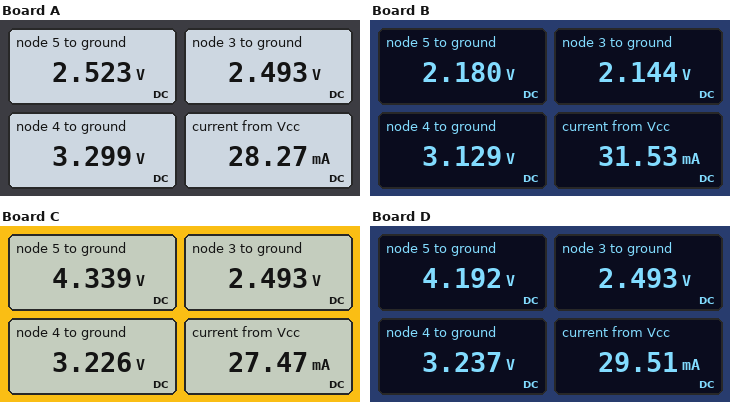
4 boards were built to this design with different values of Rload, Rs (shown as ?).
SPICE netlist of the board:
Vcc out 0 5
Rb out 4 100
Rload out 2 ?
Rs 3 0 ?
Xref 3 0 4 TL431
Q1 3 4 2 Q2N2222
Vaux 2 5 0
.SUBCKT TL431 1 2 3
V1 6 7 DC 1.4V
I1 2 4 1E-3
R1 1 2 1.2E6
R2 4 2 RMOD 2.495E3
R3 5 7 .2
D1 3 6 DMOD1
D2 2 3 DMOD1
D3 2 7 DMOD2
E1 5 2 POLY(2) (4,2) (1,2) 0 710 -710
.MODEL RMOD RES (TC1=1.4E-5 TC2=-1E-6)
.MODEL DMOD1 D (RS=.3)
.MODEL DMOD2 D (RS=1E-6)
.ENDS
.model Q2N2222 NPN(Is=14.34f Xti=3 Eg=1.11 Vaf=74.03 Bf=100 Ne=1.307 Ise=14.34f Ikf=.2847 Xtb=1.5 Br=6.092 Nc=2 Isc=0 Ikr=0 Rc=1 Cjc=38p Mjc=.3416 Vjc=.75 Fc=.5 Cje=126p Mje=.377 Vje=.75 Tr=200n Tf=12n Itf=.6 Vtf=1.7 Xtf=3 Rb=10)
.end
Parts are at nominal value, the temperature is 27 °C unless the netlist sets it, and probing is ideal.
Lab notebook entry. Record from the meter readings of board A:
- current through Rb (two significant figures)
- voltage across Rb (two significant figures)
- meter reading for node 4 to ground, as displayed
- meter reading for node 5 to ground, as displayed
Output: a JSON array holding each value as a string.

["17 mA", "1.7 V", "3.299 V", "2.523 V"]
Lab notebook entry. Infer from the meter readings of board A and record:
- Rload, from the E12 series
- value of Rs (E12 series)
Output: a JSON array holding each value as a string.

["220 Ω", "150 Ω"]
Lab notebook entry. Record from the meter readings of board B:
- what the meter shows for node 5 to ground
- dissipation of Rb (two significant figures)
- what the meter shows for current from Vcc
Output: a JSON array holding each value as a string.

["2.180 V", "35 mW", "31.53 mA"]
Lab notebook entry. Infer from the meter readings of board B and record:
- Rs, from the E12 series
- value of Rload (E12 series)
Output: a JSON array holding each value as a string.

["68 Ω", "220 Ω"]
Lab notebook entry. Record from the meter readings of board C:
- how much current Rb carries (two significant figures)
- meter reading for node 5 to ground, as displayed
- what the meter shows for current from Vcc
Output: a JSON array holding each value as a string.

["18 mA", "4.339 V", "27.47 mA"]
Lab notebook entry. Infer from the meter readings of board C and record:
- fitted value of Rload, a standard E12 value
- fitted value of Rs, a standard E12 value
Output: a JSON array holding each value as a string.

["68 Ω", "220 Ω"]
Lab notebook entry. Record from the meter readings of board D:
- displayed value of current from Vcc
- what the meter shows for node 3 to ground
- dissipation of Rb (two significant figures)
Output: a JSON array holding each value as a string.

["29.51 mA", "2.493 V", "31 mW"]
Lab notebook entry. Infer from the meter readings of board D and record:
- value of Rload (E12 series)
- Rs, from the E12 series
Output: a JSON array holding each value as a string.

["68 Ω", "180 Ω"]
